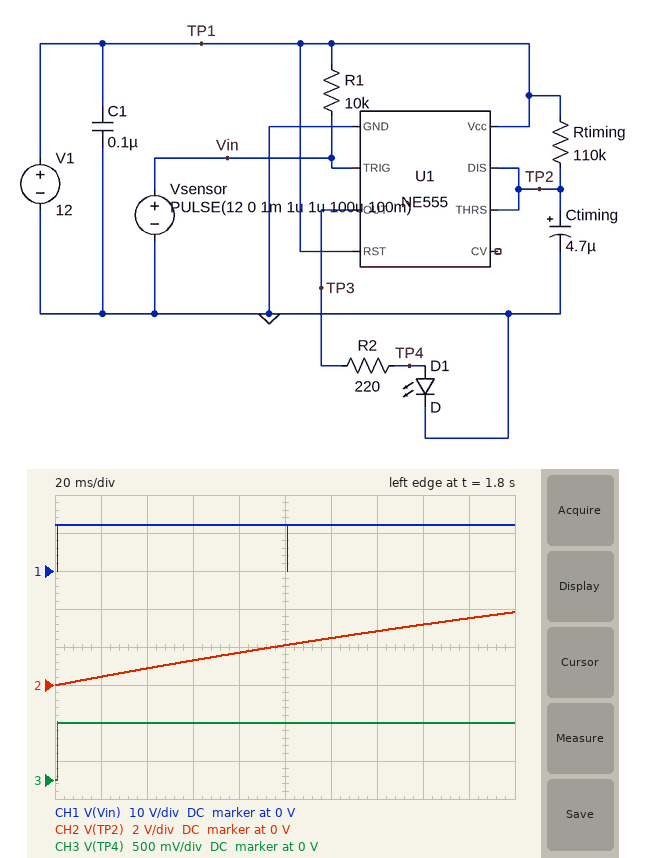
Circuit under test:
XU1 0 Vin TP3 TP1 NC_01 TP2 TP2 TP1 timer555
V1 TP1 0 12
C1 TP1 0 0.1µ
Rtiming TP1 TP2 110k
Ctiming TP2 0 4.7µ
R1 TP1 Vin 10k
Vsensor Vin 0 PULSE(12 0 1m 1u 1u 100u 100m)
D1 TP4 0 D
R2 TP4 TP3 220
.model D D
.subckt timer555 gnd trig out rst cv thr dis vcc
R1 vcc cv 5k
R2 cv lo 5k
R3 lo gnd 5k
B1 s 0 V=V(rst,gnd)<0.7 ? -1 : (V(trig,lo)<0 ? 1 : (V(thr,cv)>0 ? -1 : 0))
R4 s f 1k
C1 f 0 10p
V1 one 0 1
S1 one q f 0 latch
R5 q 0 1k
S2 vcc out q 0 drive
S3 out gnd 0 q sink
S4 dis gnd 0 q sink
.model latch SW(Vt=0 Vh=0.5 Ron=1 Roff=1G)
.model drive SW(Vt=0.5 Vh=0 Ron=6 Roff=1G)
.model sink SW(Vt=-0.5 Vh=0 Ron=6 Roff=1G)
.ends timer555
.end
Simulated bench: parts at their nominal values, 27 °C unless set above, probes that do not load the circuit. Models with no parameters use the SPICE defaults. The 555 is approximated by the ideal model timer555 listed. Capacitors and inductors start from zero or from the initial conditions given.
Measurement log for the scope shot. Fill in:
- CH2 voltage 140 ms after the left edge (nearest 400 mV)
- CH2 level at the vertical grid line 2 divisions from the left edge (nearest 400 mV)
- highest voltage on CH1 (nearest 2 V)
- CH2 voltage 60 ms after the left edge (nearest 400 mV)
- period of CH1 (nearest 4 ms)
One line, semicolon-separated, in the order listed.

2.8 V; 800 mV; 12 V; 1.2 V; 100 ms
